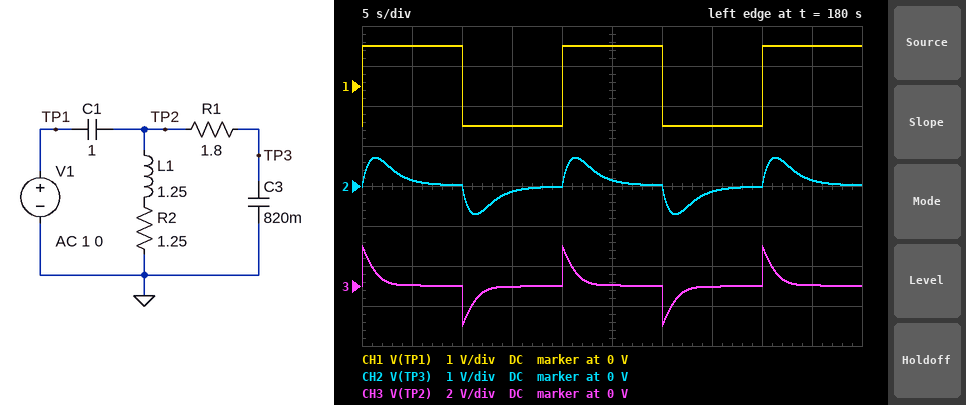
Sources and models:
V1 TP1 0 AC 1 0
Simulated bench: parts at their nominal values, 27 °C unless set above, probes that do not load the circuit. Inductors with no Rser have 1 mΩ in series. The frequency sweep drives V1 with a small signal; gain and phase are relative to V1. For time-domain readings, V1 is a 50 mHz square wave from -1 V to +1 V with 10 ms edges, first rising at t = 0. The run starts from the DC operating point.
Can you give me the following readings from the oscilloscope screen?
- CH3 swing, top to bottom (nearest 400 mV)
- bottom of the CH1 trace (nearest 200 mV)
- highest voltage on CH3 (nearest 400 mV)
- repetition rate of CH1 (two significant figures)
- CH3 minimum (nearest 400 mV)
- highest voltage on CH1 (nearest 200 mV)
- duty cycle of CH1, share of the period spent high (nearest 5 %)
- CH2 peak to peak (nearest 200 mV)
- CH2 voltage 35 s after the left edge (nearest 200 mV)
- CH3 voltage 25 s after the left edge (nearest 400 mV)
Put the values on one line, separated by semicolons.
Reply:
4.0 V; -1.0 V; 2.0 V; 50 mHz; -2.0 V; 1.0 V; 50 %; 1.4 V; -200 mV; 0 V
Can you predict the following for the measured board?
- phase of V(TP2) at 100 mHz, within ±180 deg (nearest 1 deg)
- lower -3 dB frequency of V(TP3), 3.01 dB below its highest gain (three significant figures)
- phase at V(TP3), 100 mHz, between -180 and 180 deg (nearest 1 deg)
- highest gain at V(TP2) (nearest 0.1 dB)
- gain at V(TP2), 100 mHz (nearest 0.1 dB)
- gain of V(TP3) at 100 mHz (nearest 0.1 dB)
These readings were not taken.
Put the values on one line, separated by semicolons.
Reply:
57 deg; 55.0 mHz; 14 deg; 0.2 dB; -4.0 dB; -6.7 dB
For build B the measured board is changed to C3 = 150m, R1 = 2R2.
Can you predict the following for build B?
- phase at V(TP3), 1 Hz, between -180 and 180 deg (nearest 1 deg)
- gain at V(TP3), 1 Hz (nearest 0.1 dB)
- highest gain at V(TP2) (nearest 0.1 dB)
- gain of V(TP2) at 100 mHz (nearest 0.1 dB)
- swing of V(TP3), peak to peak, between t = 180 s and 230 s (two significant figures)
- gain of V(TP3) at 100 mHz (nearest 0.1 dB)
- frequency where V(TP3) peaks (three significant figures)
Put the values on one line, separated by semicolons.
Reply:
-61 deg; -7.3 dB; 1.3 dB; -0.8 dB; 2.9 V; -1.0 dB; 158 mHz
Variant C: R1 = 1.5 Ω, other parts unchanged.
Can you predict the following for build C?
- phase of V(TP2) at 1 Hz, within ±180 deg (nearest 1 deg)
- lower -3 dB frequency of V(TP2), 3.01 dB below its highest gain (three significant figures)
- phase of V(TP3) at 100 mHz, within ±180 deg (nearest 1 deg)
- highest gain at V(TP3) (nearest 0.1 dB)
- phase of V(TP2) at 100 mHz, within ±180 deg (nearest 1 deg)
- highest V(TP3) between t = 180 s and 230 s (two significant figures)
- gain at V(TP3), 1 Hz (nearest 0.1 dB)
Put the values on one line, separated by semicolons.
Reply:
6 deg; 122 mHz; 17 deg; -5.7 dB; 54 deg; 760 mV; -17.8 dB
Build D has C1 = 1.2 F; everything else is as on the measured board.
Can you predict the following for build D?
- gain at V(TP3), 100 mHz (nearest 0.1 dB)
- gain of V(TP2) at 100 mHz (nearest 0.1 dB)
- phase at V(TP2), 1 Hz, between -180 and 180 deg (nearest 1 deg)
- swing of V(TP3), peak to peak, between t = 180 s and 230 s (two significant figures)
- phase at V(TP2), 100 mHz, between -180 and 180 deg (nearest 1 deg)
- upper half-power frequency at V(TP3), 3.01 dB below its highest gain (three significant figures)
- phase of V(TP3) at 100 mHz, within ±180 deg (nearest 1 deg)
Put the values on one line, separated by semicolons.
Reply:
-5.7 dB; -3.0 dB; 4 deg; 1.5 V; 51 deg; 273 mHz; 8 deg
